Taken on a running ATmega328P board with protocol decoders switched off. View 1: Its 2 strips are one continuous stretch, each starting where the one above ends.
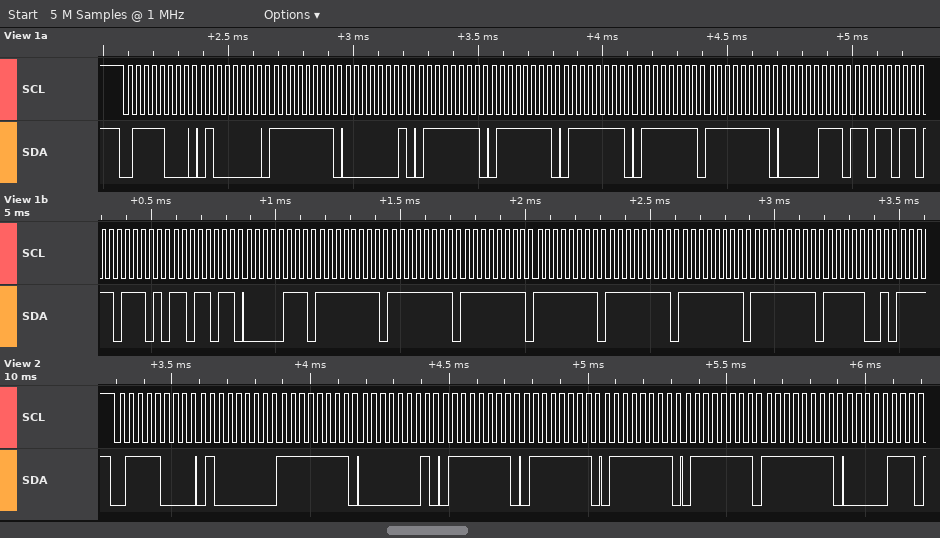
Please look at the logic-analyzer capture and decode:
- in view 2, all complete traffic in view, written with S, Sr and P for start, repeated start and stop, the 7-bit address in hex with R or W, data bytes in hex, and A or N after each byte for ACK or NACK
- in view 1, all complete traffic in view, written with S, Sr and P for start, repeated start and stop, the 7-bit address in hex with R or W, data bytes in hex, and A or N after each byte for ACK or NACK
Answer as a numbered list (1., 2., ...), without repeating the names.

1. S 3CW A 40 A FF A 01 A 7F A 7F A 7F A 7F A FF A 07 A
2. S 3CW A 40 A FF A 01 A 7F A 7F A 7F A 7F A FF A 07 A DB A DD A DB A 07 A FF A FF A FF A FF A FF A FF A FF A F9 A
